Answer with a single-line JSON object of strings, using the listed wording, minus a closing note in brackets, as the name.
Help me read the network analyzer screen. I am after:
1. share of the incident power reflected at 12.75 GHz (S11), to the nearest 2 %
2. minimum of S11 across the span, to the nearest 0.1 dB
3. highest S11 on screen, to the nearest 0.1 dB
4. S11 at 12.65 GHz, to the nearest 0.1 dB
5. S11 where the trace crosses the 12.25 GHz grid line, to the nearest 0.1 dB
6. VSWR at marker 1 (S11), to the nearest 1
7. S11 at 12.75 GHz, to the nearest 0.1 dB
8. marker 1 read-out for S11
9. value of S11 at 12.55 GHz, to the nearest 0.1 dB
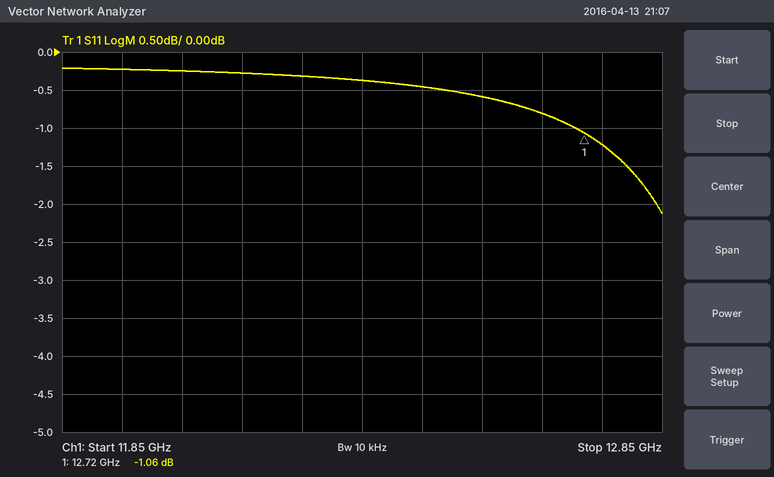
{"share of the incident power reflected at 12.75 GHz (S11), to the nearest 2 %": "76 %", "minimum of S11 across the span, to the nearest 0.1 dB": "-2.1 dB", "highest S11 on screen, to the nearest 0.1 dB": "-0.2 dB", "S11 at 12.65 GHz, to the nearest 0.1 dB": "-0.8 dB", "S11 where the trace crosses the 12.25 GHz grid line, to the nearest 0.1 dB": "-0.3 dB", "VSWR at marker 1 (S11), to the nearest 1": "16", "S11 at 12.75 GHz, to the nearest 0.1 dB": "-1.2 dB", "marker 1 read-out for S11": "-1.06 dB", "value of S11 at 12.55 GHz, to the nearest 0.1 dB": "-0.6 dB"}
